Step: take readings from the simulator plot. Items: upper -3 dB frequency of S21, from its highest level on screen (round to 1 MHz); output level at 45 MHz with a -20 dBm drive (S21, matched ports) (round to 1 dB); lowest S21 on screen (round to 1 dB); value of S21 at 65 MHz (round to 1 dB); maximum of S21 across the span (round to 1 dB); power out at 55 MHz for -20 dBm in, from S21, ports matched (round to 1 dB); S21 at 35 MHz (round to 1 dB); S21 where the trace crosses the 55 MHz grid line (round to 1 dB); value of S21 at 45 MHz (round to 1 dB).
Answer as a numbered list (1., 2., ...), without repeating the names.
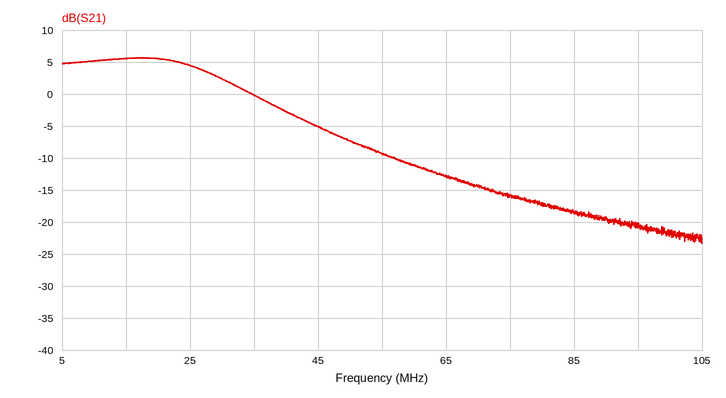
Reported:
1. 29 MHz
2. -25 dBm
3. -23 dB
4. -13 dB
5. 6 dB
6. -29 dBm
7. 0 dB
8. -9 dB
9. -5 dB
